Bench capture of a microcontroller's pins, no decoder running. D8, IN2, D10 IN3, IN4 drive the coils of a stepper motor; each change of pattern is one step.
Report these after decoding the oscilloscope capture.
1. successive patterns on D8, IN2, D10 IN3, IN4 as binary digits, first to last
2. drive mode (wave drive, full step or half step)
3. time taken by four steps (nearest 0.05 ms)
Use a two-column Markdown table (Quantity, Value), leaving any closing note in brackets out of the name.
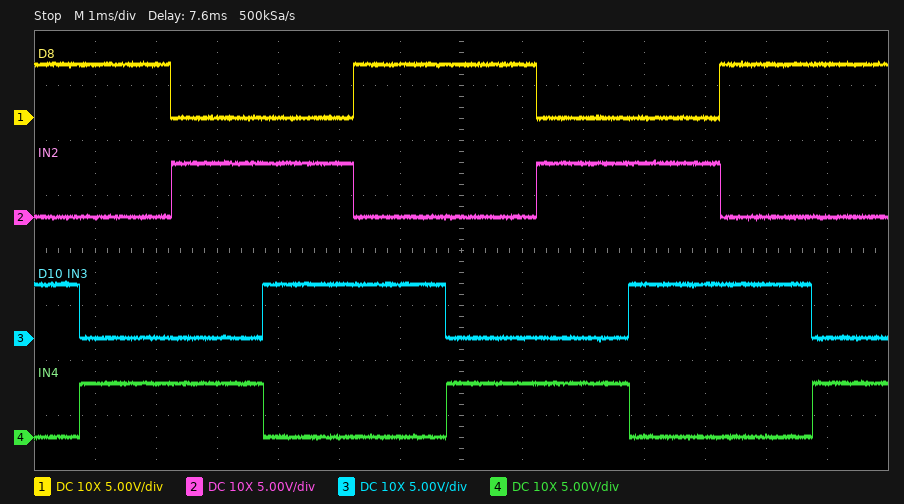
| Quantity | Value |
|---|---|
| successive patterns on D8, IN2, D10 IN3, IN4 as binary digits, first to last | 1010 1001 0101 0110 1010 1001 0101 0110 1010 1001 |
| drive mode | full step |
| time taken by four steps | 6.00 ms |
